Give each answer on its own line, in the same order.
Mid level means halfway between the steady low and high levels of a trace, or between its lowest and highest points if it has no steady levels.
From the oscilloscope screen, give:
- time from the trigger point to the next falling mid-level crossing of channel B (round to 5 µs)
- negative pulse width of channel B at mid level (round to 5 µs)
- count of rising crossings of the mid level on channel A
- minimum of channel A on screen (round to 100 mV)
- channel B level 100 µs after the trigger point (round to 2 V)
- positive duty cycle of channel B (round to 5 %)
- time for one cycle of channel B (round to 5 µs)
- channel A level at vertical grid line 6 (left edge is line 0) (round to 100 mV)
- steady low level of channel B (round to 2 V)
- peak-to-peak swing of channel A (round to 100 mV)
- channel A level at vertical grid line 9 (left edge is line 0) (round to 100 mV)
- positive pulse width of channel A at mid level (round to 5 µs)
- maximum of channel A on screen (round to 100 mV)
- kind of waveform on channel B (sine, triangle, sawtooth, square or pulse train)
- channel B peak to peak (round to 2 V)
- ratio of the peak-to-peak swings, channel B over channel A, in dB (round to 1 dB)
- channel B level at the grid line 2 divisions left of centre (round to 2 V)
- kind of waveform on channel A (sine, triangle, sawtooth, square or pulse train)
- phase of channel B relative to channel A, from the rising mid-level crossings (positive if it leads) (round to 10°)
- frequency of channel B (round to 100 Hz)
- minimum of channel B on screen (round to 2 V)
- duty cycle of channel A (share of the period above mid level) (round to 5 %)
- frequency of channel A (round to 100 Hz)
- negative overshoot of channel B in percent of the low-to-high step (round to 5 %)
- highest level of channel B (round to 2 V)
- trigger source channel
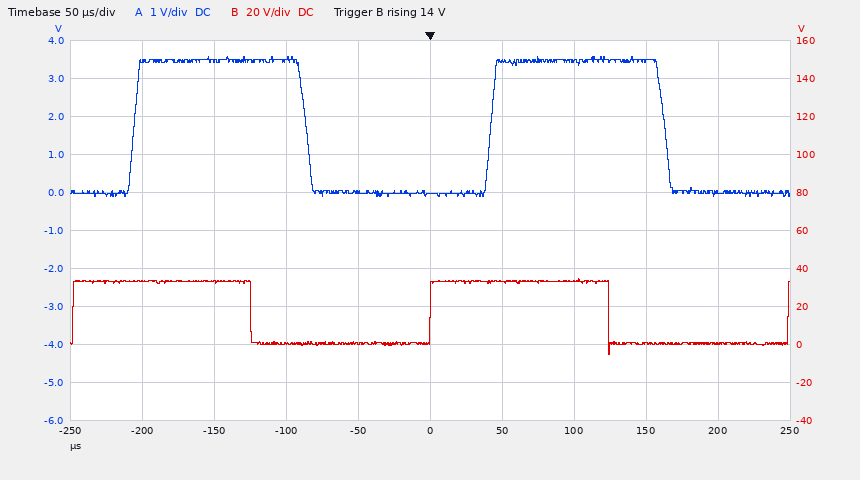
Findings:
125 µs
125 µs
2
-100 mV
34 V
50 %
250 µs
3.5 V
0 V
3.7 V
0.0 V
120 µs
3.6 V
square
40 V
21 dB
0 V
square
+60°
4.0 kHz
-6 V
50 %
4.0 kHz
20 %
34 V
channel B
